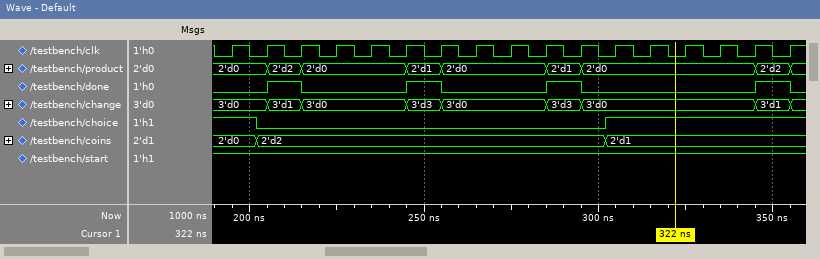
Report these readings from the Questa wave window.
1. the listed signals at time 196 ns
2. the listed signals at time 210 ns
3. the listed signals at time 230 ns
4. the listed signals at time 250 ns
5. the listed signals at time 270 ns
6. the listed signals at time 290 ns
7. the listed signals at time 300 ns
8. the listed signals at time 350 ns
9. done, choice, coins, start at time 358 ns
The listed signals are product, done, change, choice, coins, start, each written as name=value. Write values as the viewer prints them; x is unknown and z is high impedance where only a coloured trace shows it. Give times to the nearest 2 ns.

product=2'd0, done=0, change=3'd0, choice=1, coins=2'd0, start=1
product=2'd2, done=1, change=3'd1, choice=0, coins=2'd2, start=1
product=2'd0, done=0, change=3'd0, choice=0, coins=2'd2, start=1
product=2'd1, done=1, change=3'd3, choice=0, coins=2'd2, start=1
product=2'd0, done=0, change=3'd0, choice=0, coins=2'd2, start=1
product=2'd1, done=1, change=3'd3, choice=0, coins=2'd2, start=1
product=2'd0, done=0, change=3'd0, choice=0, coins=2'd2, start=1
product=2'd2, done=1, change=3'd1, choice=1, coins=2'd1, start=1
done=0, choice=1, coins=2'd1, start=1
